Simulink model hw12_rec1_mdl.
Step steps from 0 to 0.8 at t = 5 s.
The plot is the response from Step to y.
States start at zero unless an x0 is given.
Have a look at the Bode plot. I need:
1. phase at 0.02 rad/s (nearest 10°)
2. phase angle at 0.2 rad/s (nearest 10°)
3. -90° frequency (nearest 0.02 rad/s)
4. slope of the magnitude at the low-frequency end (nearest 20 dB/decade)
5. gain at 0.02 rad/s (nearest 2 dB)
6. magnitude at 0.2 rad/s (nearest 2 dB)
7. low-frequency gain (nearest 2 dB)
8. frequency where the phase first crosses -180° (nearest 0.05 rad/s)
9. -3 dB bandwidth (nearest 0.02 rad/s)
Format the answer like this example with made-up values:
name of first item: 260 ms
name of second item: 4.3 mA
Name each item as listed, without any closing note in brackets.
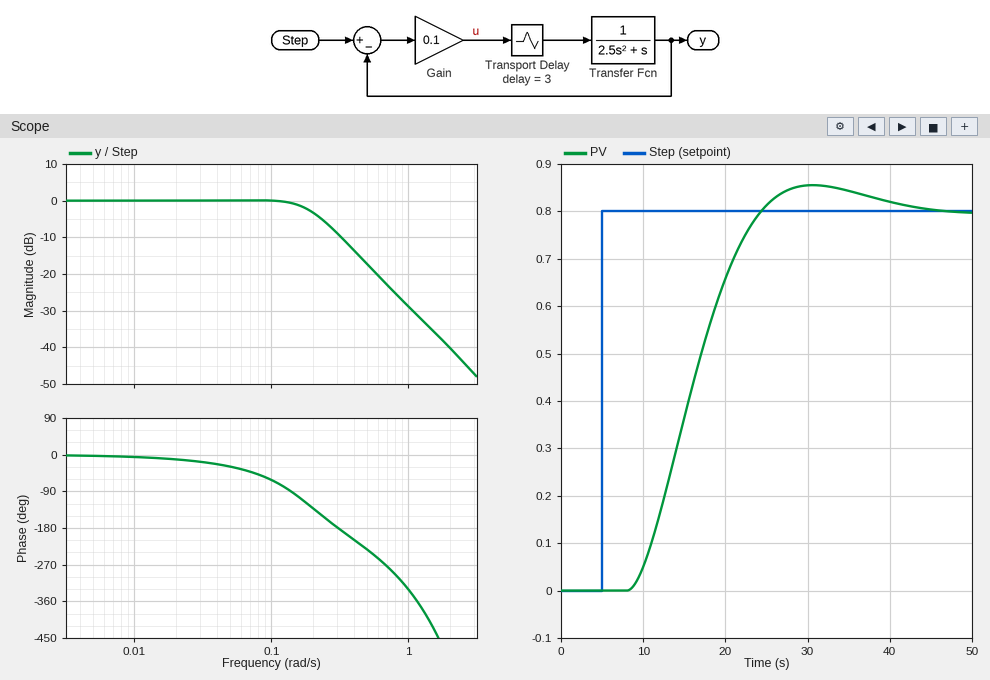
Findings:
phase at 0.02 rad/s: -10°
phase angle at 0.2 rad/s: -130°
-90° frequency: 0.14 rad/s
slope of the magnitude at the low-frequency end: 0 dB/decade
gain at 0.02 rad/s: 0 dB
magnitude at 0.2 rad/s: -4 dB
low-frequency gain: 0 dB
frequency where the phase first crosses -180°: 0.30 rad/s
-3 dB bandwidth: 0.20 rad/s
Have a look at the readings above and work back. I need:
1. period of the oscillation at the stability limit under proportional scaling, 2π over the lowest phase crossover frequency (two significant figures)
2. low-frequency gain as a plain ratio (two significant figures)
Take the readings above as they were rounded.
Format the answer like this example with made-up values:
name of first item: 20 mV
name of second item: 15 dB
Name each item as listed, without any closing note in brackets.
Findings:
period of the oscillation at the stability limit under proportional scaling, 2π over the lowest phase crossover frequency: 21 s
low-frequency gain as a plain ratio: 1.0
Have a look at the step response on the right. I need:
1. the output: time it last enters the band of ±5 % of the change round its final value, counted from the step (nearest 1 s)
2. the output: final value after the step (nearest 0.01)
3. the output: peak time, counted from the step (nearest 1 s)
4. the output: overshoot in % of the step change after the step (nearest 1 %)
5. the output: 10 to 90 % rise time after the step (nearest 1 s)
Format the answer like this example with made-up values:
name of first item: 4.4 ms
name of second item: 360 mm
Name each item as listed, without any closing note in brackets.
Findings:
the output: time it last enters the band of ±5 % of the change round its final value, counted from the step: 31 s
the output: final value after the step: 0.80
the output: peak time, counted from the step: 26 s
the output: overshoot in % of the step change after the step: 7 %
the output: 10 to 90 % rise time after the step: 11 s
